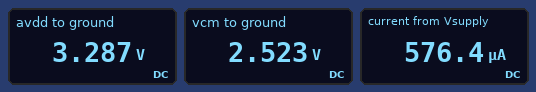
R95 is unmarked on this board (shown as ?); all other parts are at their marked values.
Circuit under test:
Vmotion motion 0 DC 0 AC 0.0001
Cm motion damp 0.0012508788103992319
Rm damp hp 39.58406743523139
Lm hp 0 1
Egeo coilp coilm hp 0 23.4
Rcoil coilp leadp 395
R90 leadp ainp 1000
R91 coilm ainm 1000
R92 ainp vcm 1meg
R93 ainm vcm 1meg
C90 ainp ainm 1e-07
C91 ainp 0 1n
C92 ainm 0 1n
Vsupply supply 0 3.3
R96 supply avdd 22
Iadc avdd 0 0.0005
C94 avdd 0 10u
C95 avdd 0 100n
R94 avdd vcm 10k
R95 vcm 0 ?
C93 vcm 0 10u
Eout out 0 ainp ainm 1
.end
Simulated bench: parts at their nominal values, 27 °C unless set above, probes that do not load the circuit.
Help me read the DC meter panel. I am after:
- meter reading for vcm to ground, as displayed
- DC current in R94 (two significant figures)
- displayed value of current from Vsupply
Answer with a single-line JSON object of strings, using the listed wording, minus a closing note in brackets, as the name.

{"meter reading for vcm to ground, as displayed": "2.523 V", "DC current in R94": "76 µA", "displayed value of current from Vsupply": "576.4 µA"}
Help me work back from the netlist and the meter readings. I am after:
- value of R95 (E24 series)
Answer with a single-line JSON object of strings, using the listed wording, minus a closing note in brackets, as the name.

{"value of R95": "33 kΩ"}
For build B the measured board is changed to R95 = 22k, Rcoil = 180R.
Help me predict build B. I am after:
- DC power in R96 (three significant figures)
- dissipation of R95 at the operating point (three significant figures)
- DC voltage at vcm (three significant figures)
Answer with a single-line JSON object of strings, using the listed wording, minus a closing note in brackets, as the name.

{"DC power in R96": "7.99 µW", "dissipation of R95 at the operating point": "232 µW", "DC voltage at vcm": "2.26 V"}
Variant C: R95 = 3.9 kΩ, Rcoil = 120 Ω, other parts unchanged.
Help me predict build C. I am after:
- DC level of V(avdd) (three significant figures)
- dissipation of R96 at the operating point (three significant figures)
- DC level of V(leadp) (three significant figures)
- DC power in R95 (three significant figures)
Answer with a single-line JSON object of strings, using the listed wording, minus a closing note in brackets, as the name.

{"DC level of V(avdd)": "3.28 V", "dissipation of R96 at the operating point": "11.9 µW", "DC level of V(leadp)": "921 mV", "DC power in R95": "218 µW"}
